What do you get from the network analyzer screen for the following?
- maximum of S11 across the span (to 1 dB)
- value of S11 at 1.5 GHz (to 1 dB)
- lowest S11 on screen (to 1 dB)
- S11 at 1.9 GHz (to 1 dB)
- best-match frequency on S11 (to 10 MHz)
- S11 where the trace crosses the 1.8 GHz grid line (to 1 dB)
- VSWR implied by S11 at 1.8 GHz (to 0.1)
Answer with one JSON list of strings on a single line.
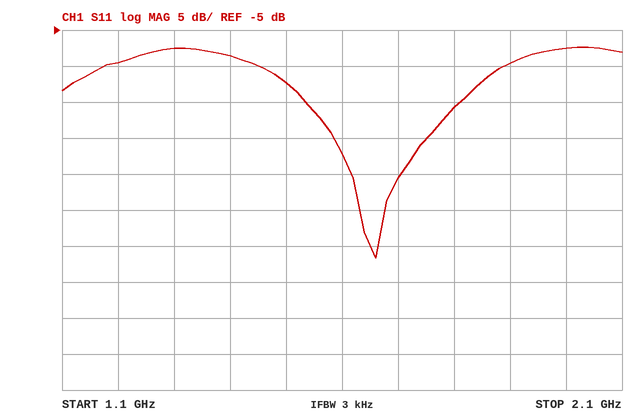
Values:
["-7 dB", "-12 dB", "-37 dB", "-10 dB", "1.66 GHz", "-16 dB", "1.4"]
